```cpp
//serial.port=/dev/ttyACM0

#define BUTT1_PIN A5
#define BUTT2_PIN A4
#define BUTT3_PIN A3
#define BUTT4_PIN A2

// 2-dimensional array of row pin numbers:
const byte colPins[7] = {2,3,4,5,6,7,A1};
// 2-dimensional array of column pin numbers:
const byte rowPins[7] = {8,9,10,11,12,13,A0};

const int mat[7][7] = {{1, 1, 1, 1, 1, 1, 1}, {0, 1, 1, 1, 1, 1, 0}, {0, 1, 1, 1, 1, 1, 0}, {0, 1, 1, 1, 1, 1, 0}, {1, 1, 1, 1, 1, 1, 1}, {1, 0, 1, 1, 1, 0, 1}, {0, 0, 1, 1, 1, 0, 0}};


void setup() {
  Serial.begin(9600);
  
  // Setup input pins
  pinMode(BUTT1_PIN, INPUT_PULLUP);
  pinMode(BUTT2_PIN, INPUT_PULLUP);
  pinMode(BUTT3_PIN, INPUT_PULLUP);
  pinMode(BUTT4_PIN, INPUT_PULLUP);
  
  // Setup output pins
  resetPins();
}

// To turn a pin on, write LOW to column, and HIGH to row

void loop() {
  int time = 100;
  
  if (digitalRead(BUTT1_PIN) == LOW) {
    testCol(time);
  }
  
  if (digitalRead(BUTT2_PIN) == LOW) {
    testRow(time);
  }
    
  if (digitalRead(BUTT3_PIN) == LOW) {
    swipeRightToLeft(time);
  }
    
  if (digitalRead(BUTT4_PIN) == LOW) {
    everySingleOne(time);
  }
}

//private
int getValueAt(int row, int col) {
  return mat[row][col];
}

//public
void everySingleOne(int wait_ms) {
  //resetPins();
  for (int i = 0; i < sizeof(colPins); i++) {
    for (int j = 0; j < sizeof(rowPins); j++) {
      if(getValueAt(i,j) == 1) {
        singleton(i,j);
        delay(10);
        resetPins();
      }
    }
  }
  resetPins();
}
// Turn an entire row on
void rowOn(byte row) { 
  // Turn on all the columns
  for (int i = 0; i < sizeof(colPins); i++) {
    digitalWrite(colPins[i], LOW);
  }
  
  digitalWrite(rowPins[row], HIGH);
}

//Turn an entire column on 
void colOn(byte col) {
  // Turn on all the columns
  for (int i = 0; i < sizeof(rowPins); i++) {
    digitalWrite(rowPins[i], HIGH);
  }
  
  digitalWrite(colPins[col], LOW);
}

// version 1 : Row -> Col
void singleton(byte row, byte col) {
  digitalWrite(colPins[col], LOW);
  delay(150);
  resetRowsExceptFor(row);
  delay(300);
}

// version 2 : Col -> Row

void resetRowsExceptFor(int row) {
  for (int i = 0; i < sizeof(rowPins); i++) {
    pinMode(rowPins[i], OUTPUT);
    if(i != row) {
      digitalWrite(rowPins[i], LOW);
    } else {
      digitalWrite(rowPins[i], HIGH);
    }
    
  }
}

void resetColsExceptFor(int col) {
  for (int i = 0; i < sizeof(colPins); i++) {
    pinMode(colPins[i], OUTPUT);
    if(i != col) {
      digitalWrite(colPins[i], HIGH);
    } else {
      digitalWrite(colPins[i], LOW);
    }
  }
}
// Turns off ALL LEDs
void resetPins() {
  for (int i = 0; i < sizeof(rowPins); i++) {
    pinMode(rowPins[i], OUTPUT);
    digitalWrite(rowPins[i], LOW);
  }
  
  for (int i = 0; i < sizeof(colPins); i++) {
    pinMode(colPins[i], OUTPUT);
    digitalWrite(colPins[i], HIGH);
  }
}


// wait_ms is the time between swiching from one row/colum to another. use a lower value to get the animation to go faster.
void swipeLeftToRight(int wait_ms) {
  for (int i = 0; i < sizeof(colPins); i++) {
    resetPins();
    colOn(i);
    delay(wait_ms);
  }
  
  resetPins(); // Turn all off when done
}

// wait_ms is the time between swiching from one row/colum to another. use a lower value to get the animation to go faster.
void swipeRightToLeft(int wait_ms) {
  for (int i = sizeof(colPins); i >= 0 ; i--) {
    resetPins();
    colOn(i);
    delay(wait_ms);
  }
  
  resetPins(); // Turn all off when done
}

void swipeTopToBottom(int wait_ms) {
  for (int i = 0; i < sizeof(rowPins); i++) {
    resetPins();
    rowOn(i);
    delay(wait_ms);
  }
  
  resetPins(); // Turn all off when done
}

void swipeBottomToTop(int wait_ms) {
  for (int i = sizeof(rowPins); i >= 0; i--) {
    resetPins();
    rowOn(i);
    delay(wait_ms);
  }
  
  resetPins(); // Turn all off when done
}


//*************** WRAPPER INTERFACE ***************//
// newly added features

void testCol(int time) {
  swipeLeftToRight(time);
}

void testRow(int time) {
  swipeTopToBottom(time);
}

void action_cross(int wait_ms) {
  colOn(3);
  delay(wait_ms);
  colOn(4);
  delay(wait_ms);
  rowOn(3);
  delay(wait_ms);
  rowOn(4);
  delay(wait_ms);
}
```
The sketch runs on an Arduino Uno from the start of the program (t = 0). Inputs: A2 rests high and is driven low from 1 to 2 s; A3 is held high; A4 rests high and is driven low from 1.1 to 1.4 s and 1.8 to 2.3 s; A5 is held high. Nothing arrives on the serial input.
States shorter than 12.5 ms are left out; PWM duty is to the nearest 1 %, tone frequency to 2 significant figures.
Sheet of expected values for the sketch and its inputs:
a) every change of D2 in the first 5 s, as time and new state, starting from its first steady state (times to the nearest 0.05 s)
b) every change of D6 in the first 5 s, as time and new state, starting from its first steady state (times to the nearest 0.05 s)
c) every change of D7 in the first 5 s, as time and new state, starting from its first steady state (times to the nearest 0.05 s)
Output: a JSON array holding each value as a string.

["0 s high; 1 s low; 1.45 s high", "0 s high; 2.85 s low; 3.3 s high", "0 s high; 3.3 s low; 3.75 s high"]
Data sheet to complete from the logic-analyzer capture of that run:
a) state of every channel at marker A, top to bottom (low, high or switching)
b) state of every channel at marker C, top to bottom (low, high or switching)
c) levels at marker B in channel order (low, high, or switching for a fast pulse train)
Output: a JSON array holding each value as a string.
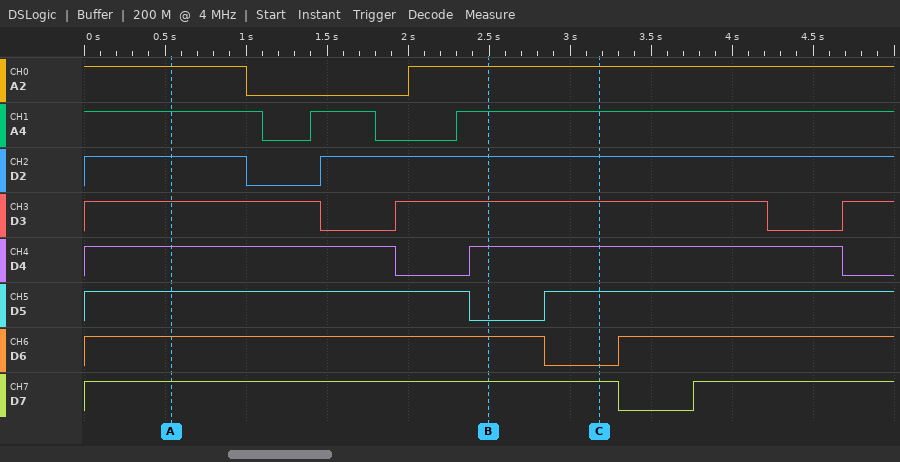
["A2 high, A4 high, D2 high, D3 high, D4 high, D5 high, D6 high, D7 high", "A2 high, A4 high, D2 high, D3 high, D4 high, D5 high, D6 low, D7 high", "A2 high, A4 high, D2 high, D3 high, D4 high, D5 low, D6 high, D7 high"]
